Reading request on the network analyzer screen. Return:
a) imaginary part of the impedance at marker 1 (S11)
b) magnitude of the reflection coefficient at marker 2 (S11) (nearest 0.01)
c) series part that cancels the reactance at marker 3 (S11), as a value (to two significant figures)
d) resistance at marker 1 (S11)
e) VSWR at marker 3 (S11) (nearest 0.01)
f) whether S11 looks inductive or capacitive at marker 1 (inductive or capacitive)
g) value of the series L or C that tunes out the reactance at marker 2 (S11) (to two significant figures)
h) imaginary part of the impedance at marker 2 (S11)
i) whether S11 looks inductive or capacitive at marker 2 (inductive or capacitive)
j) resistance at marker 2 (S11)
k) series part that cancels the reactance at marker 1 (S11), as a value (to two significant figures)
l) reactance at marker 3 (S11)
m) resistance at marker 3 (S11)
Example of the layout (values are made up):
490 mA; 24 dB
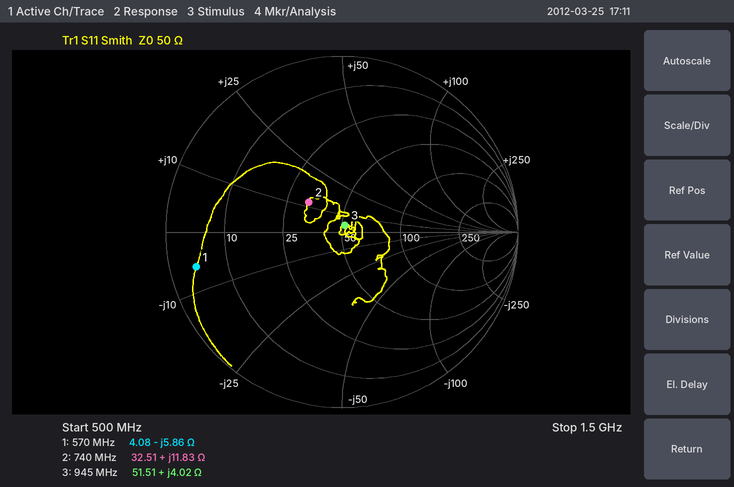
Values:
-5.86 Ω; 0.25; 42 pF; 4.08 Ω; 1.09; capacitive; 18 pF; +11.83 Ω; inductive; 32.51 Ω; 1.6 nH; +4.02 Ω; 51.51 Ω
